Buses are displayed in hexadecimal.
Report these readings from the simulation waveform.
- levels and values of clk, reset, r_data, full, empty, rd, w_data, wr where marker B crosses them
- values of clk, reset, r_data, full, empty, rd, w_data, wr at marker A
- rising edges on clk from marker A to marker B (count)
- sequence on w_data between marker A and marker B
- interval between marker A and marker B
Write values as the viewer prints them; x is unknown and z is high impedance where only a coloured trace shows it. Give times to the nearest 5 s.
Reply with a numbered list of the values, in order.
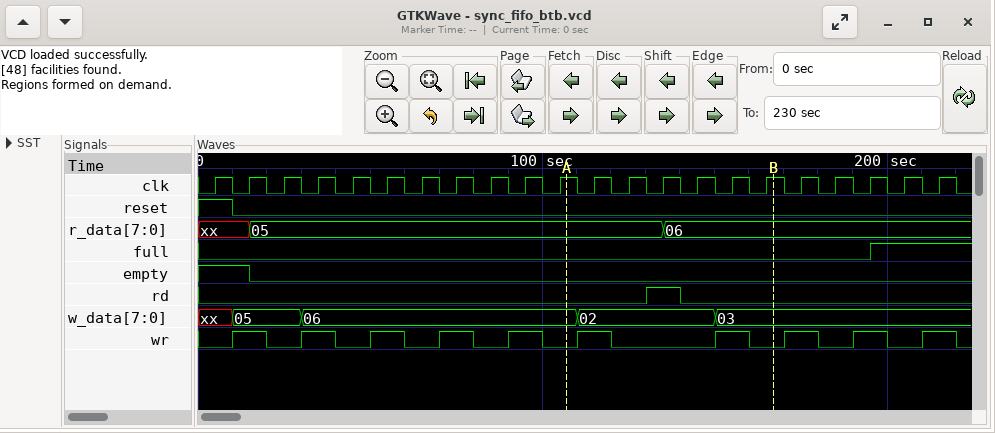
1. clk=1, reset=0, r_data=06, full=0, empty=0, rd=0, w_data=03, wr=0
2. clk=1, reset=0, r_data=05, full=0, empty=0, rd=0, w_data=06, wr=0
3. 6
4. 06, 02, 03
5. 60 s
